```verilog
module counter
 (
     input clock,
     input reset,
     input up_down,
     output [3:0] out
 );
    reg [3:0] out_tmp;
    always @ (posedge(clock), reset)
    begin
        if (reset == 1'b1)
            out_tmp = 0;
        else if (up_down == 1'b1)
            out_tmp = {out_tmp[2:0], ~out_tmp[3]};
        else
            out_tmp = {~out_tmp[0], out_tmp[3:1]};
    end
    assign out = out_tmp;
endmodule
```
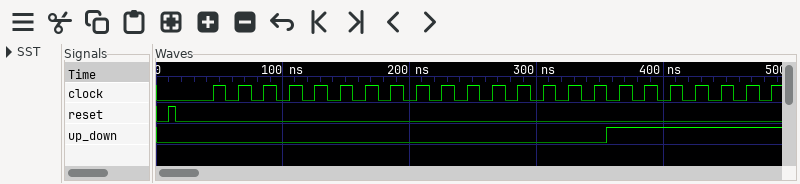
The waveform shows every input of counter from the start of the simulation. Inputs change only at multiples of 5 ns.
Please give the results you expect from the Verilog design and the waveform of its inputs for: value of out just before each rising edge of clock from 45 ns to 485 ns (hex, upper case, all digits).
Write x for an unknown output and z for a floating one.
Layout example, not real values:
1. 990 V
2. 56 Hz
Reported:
1. 8, C, E, F, 7, 3, 1, 0, 8, C, E, F, 7, 3, 1, 0, 8, 0, 1, 3, 7, F, E
